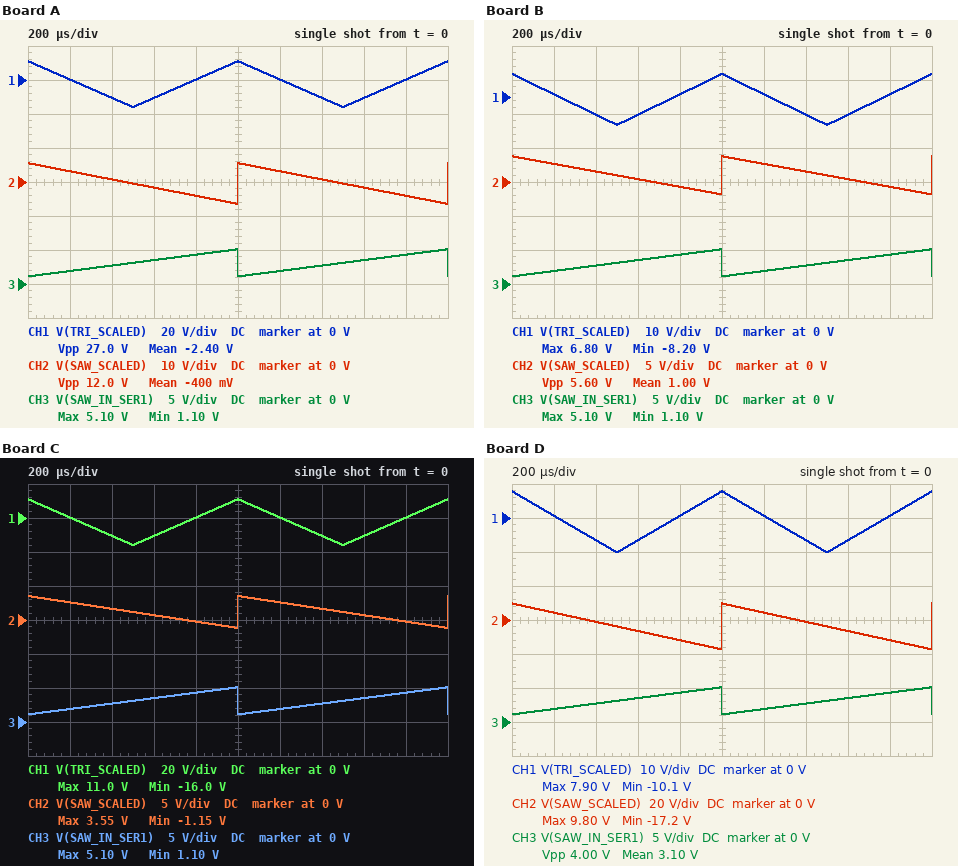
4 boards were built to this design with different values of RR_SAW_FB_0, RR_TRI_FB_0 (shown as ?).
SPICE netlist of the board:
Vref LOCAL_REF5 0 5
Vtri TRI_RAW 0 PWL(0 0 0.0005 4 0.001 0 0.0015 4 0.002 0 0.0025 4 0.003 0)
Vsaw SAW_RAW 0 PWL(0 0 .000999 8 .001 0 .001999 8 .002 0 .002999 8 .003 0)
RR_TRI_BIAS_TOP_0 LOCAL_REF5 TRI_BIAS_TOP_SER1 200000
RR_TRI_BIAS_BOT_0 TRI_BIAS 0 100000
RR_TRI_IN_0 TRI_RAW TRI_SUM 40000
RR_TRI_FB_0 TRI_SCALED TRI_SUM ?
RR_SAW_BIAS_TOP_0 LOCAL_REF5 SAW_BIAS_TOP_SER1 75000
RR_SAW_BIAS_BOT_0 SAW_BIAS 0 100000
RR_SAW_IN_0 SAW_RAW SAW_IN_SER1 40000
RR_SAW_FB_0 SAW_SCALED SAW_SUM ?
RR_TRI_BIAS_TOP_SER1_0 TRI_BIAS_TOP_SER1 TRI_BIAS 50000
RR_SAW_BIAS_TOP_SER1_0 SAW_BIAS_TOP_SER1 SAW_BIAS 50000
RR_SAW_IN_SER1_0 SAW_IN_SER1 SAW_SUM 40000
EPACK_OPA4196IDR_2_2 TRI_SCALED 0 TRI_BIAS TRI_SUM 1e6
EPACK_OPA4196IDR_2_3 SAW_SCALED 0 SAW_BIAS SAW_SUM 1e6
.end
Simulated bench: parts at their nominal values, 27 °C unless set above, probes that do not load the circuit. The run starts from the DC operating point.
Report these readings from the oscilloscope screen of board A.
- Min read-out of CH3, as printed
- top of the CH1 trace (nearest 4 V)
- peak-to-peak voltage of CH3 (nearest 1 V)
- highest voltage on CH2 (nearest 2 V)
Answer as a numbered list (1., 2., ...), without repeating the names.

1. 1.10 V
2. 12 V
3. 4 V
4. 6 V
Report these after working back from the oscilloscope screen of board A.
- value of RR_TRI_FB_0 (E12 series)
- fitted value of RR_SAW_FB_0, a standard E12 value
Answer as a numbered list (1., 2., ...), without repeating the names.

1. 270 kΩ
2. 120 kΩ
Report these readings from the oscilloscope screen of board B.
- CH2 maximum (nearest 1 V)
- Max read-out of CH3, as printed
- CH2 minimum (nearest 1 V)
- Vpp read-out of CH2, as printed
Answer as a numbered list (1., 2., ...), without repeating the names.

1. 4 V
2. 5.10 V
3. -2 V
4. 5.60 V
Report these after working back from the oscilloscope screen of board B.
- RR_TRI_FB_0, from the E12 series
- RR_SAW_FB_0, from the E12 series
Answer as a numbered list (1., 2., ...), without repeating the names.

1. 150 kΩ
2. 56 kΩ
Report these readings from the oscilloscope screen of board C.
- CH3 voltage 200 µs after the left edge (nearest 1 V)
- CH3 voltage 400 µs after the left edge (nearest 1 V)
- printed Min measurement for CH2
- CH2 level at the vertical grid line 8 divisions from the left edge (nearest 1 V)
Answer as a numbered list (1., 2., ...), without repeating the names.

1. 2 V
2. 3 V
3. -1.15 V
4. 1 V
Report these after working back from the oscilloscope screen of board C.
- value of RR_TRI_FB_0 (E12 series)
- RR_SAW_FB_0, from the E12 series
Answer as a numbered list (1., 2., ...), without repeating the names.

1. 270 kΩ
2. 47 kΩ
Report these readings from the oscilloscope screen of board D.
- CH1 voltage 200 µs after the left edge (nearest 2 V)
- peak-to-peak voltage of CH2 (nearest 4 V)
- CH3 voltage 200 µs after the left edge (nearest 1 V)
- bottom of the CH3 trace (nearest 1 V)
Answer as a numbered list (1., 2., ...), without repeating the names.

1. 0 V
2. 28 V
3. 2 V
4. 1 V
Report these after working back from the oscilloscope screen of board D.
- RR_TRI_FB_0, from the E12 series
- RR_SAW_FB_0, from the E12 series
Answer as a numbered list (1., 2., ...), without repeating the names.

1. 180 kΩ
2. 270 kΩ
